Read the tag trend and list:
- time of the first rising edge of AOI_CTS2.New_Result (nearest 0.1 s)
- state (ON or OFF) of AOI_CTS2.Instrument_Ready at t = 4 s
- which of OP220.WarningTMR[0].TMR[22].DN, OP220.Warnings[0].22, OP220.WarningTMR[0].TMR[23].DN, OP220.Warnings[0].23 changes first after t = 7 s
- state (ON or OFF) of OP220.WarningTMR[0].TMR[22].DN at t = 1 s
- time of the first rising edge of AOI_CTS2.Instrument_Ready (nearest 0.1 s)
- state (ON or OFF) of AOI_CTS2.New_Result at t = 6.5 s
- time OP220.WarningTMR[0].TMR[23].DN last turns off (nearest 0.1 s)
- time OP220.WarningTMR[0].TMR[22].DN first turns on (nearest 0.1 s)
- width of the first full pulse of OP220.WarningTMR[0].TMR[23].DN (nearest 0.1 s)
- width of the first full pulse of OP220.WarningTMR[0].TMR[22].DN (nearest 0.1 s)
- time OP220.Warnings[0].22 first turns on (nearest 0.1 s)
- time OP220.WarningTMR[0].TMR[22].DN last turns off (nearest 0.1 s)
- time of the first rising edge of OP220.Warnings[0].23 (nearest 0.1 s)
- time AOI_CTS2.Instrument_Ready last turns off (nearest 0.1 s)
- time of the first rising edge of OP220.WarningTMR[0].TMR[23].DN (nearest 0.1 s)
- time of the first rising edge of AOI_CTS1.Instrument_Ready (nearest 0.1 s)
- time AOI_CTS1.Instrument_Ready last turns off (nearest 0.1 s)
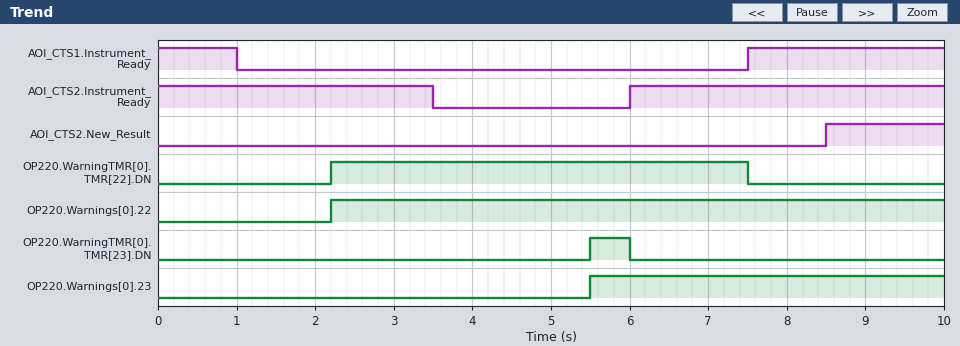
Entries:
8.5 s
OFF
OP220.WarningTMR[0].TMR[22].DN
OFF
6.0 s
OFF
6.0 s
2.2 s
0.5 s
5.3 s
2.2 s
7.5 s
5.5 s
3.5 s
5.5 s
7.5 s
1.0 s
